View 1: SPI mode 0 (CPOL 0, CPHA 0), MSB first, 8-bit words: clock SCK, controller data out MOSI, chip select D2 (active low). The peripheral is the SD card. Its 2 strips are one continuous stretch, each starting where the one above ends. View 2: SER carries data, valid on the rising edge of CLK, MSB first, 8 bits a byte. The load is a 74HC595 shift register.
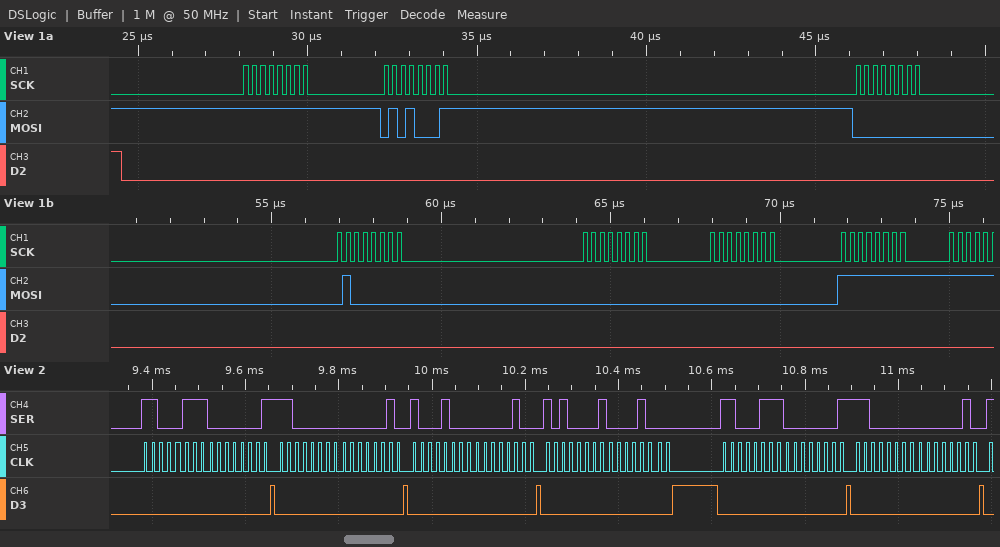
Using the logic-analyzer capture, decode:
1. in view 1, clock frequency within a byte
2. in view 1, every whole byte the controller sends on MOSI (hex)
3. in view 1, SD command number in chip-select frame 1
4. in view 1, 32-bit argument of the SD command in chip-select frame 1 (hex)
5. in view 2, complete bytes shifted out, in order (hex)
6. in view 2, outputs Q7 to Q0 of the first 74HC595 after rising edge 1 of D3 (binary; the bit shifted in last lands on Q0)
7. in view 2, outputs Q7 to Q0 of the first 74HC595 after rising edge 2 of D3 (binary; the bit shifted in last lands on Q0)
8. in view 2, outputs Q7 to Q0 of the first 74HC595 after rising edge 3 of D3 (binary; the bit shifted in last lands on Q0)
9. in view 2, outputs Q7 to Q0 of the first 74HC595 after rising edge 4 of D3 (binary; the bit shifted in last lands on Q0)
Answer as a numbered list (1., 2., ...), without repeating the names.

1. 4 MHz
2. FF 51 00 40 00 00 FF
3. CMD17
4. 0x00400000
5. 0xC7 0x01 0xC0 0x02 0x88 0x04 0xA1 0x08 0xC7 0x01 0xC0 0x02
6. 00000001
7. 00000010
8. 00000100
9. 00001000
